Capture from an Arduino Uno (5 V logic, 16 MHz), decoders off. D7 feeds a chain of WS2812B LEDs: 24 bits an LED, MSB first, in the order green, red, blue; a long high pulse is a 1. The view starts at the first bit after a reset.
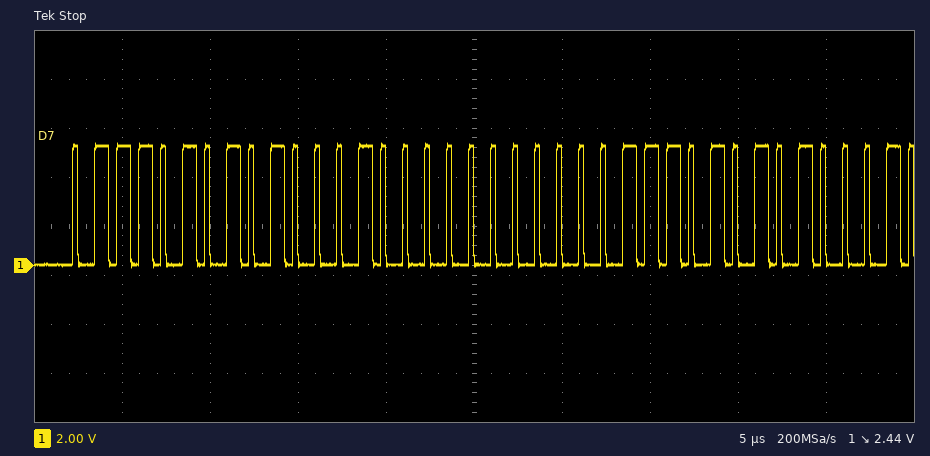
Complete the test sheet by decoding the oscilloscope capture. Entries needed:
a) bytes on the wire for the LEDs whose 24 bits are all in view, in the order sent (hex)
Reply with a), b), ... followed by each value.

a) 75 44 00
